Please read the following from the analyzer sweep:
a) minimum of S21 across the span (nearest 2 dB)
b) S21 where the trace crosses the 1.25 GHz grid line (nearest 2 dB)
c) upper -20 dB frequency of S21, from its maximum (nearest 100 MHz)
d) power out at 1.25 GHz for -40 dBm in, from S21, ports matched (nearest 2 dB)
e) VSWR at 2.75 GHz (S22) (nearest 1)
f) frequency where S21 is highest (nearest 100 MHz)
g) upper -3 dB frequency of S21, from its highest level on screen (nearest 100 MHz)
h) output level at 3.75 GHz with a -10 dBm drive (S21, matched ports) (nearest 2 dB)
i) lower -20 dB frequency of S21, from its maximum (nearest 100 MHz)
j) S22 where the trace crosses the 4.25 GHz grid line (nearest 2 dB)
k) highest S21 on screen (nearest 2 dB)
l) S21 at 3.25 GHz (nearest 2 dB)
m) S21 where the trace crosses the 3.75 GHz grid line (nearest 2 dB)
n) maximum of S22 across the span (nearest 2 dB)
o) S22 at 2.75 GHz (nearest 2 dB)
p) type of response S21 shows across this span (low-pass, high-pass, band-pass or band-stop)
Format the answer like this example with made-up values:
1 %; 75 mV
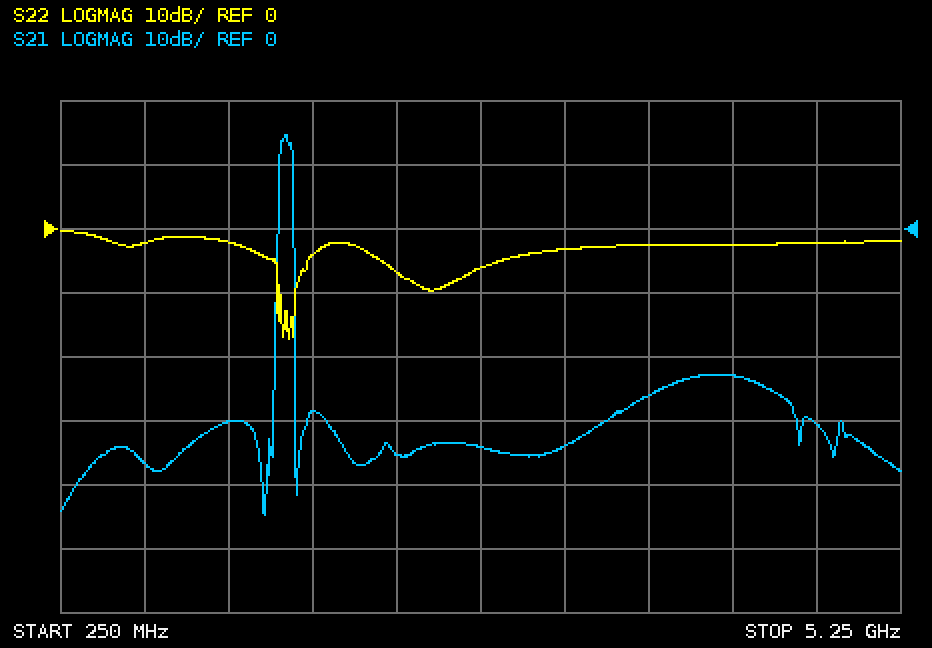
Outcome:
-44 dB; -30 dB; 1.6 GHz; -70 dBm; 3; 1.6 GHz; 1.6 GHz; -36 dBm; 1.5 GHz; -2 dB; 14 dB; -34 dB; -26 dB; 0 dB; -6 dB; band-pass
